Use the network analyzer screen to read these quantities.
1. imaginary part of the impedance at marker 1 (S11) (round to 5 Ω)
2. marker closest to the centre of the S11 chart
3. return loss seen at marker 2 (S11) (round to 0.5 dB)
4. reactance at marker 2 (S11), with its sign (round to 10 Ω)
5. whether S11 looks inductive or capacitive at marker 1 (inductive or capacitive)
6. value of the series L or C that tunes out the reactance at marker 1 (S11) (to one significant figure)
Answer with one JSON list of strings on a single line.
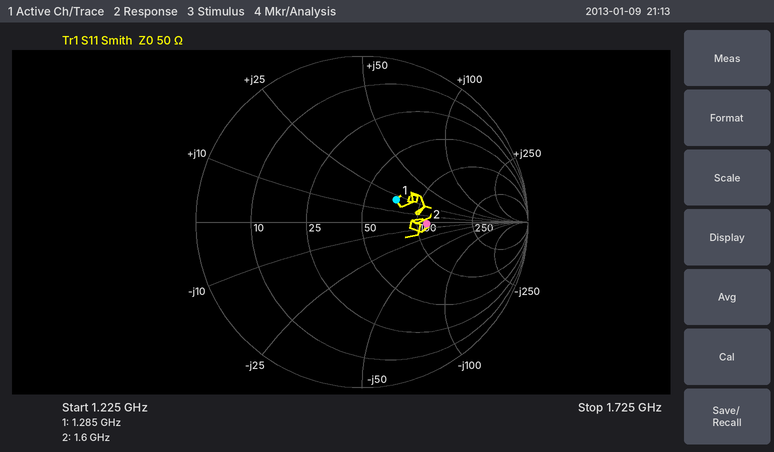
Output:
["+20 Ω", "marker 1", "8.0 dB", "0 Ω", "inductive", "6 pF"]
